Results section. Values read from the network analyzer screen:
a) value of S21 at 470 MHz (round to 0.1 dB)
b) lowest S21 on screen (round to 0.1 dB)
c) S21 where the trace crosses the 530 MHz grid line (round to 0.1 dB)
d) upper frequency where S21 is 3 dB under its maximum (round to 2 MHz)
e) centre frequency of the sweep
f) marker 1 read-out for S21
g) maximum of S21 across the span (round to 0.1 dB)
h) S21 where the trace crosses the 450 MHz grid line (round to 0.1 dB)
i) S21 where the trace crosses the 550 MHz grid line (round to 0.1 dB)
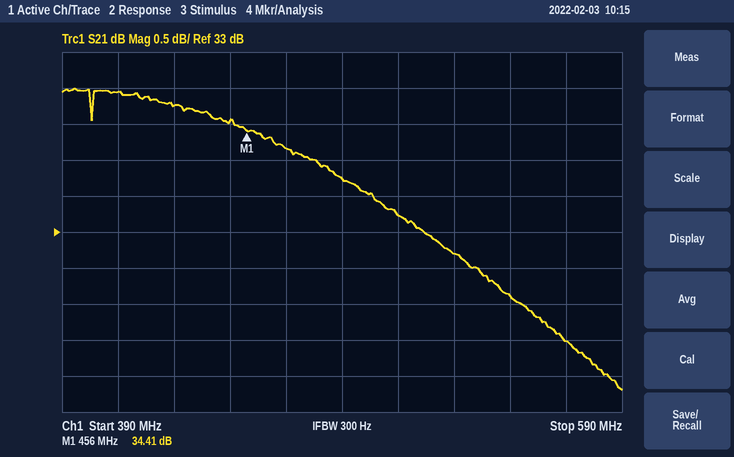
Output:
34.2 dB
30.8 dB
32.7 dB
554 MHz
490 MHz
34.41 dB
35.0 dB
34.5 dB
32.1 dB
